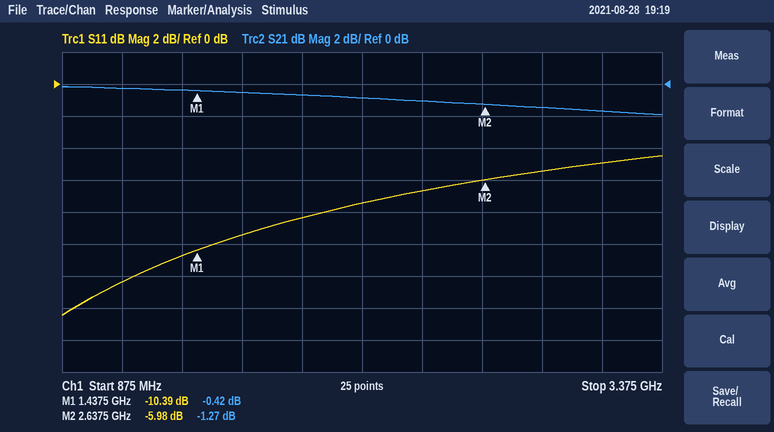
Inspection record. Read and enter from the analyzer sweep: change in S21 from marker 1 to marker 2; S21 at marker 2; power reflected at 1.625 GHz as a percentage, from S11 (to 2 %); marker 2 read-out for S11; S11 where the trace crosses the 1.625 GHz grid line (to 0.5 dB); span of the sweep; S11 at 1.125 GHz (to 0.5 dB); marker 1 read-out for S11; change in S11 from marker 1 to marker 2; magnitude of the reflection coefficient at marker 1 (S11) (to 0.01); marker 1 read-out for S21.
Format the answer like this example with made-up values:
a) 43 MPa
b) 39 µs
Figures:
a) -0.85 dB
b) -1.27 dB
c) 12 %
d) -5.98 dB
e) -9.5 dB
f) 2.5 GHz
g) -12.5 dB
h) -10.39 dB
i) 4.41 dB
j) 0.30
k) -0.42 dB
